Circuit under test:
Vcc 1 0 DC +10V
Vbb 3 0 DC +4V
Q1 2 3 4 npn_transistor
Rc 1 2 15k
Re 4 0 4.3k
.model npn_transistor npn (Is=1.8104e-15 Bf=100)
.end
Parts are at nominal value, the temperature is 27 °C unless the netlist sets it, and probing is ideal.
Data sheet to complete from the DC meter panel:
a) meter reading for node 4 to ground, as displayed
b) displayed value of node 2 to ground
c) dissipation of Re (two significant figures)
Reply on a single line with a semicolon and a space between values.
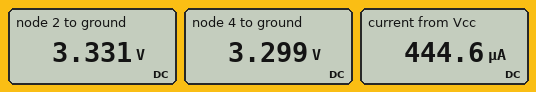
3.299 V; 3.331 V; 2.5 mW
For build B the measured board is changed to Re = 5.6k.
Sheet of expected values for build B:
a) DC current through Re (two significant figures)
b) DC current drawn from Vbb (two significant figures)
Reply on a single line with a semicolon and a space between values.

590 µA; 150 µA
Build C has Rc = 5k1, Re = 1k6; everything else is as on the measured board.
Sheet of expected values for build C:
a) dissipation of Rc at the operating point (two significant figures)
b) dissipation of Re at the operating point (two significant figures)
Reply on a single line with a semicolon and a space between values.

8.8 mW; 6.7 mW
